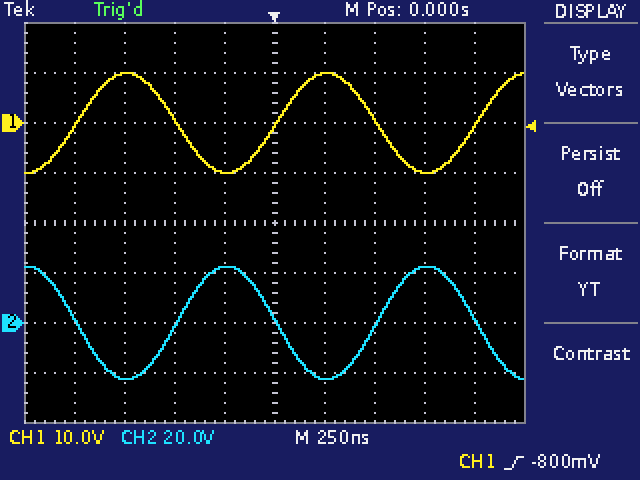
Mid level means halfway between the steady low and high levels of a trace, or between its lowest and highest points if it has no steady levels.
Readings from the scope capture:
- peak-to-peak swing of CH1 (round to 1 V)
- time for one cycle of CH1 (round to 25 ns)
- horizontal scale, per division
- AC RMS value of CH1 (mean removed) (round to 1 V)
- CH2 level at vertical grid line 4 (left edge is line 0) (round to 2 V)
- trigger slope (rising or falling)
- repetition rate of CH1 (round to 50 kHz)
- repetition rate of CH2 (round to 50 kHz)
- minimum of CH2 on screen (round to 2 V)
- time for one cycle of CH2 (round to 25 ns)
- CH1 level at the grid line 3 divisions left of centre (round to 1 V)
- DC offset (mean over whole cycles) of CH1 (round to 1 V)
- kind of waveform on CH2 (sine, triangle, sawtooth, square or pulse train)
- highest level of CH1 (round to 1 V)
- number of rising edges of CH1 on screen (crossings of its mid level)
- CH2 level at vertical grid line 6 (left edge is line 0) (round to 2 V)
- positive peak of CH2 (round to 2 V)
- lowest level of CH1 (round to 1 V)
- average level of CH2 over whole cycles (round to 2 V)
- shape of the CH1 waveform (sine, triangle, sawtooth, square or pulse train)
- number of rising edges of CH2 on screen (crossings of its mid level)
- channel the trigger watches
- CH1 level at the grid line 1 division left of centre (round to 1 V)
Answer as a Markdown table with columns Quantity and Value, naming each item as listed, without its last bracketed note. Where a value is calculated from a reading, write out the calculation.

| Quantity | Value |
|---|---|
| peak-to-peak swing of CH1 | 10 V − (-10 V) = 20 V |
| time for one cycle of CH1 | 1.000 µs |
| horizontal scale, per division | 250 ns |
| AC RMS value of CH1 (mean removed) | 20 V / (2√2) ≈ 7 V |
| CH2 level at vertical grid line 4 (left edge is line 0) | 22 V |
| trigger slope | rising |
| repetition rate of CH1 | 1 / 1.000 µs ≈ 1.00 MHz |
| repetition rate of CH2 | 1 / 1.000 µs ≈ 1.00 MHz |
| minimum of CH2 on screen | -22 V |
| time for one cycle of CH2 | 1.000 µs |
| CH1 level at the grid line 3 divisions left of centre | 10 V |
| DC offset (mean over whole cycles) of CH1 | (10 V + (-10 V)) / 2 ≈ 0 V |
| kind of waveform on CH2 | sine |
| highest level of CH1 | 10 V |
| number of rising edges of CH1 on screen | 3 |
| CH2 level at vertical grid line 6 (left edge is line 0) | -22 V |
| positive peak of CH2 | 22 V |
| lowest level of CH1 | -10 V |
| average level of CH2 over whole cycles | (22 V + (-22 V)) / 2 ≈ 0 V |
| shape of the CH1 waveform | sine |
| number of rising edges of CH2 on screen | 2 |
| channel the trigger watches | CH1 |
| CH1 level at the grid line 1 division left of centre | -10 V |
